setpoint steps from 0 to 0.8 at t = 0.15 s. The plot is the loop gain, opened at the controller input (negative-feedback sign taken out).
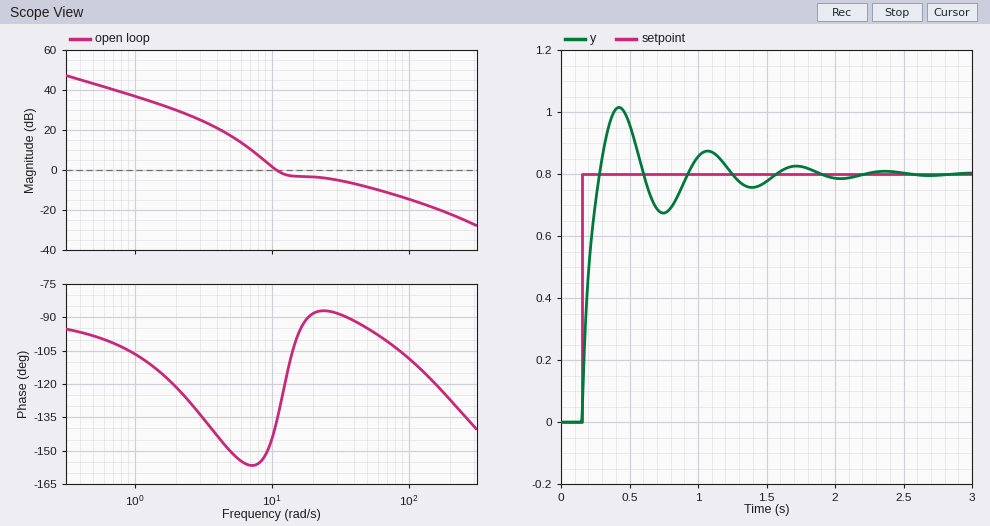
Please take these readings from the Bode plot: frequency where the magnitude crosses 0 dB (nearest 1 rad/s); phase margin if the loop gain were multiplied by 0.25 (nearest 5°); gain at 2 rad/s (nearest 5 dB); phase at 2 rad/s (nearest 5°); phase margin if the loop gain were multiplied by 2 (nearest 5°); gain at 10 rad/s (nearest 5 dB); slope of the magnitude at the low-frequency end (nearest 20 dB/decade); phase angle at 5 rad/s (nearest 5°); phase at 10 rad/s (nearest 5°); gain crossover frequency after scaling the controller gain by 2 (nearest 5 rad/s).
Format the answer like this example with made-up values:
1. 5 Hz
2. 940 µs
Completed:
1. 11 rad/s
2. 25°
3. 30 dB
4. -120°
5. 90°
6. 0 dB
7. -20 dB/decade
8. -150°
9. -145°
10. 35 rad/s
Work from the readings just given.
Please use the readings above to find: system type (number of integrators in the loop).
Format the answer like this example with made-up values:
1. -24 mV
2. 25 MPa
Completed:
1. 1
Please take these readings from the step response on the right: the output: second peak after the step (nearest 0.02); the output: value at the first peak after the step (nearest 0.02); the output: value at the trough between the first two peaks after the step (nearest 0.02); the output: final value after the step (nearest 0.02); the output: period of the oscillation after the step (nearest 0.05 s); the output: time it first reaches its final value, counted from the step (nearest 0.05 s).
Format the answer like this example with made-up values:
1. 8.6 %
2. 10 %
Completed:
1. 0.88
2. 1.02
3. 0.68
4. 0.80
5. 0.65 s
6. 0.15 s
